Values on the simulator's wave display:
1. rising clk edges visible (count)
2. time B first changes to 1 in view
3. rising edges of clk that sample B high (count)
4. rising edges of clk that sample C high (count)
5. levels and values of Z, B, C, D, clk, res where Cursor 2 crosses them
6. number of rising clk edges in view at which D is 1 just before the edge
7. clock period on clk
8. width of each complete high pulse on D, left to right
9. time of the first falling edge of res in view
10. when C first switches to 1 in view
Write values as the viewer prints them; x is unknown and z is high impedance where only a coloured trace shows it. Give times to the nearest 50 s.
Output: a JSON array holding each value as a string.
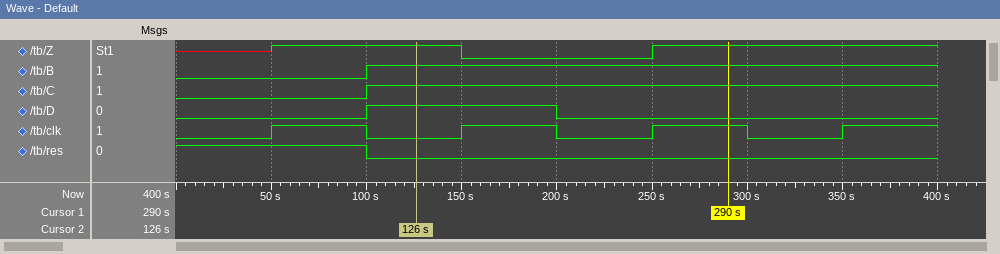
["4", "100 s", "3", "3", "Z=1, B=1, C=1, D=1, clk=0, res=0", "1", "100 s", "100 s", "100 s", "100 s"]
